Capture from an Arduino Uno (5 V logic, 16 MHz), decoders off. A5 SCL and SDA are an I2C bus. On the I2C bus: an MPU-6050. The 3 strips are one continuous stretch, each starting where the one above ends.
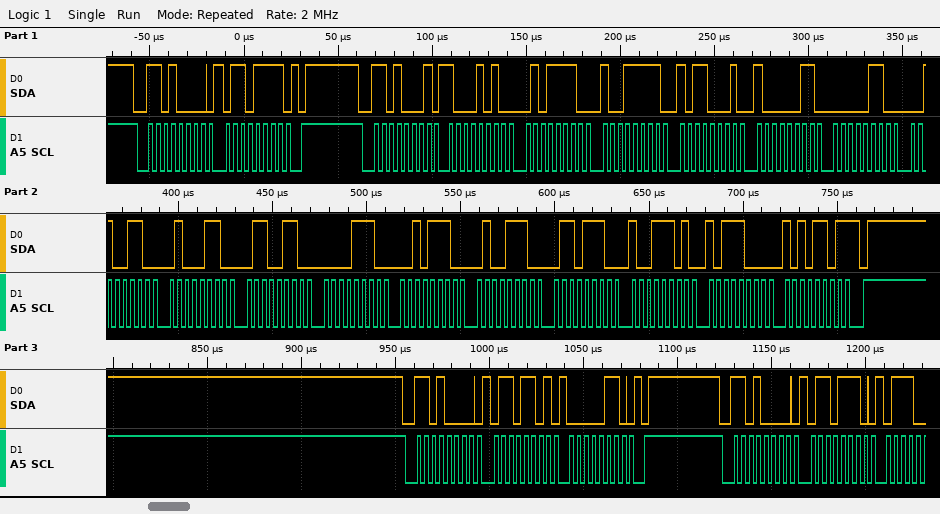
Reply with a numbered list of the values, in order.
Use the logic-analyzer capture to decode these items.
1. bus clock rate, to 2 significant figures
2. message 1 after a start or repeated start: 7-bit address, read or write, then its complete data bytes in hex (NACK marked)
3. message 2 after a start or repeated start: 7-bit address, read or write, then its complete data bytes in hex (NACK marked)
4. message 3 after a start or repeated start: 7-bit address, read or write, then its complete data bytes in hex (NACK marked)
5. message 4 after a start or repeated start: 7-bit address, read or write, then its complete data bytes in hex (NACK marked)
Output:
1. 250 kHz
2. 0x68 write: 6F
3. 0x68 read: 8A 5E 9F B1 83 06 26 46 66 0E 2E 4E 6E 9D B8 AD NACK
4. 0x68 write: 6D 06
5. 0x68 write: 6E
